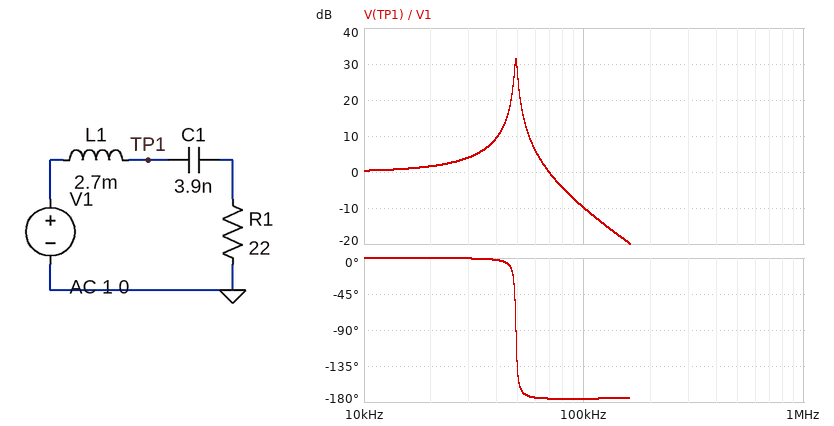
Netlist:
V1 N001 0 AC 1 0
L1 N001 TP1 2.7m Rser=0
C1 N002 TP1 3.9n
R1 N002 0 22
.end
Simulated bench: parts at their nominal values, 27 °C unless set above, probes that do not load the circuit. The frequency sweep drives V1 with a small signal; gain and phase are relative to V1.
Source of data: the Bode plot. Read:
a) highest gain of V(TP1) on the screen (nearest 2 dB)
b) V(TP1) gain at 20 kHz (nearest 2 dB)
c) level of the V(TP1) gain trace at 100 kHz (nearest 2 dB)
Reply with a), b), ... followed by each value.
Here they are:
a) 32 dB
b) 2 dB
c) -10 dB
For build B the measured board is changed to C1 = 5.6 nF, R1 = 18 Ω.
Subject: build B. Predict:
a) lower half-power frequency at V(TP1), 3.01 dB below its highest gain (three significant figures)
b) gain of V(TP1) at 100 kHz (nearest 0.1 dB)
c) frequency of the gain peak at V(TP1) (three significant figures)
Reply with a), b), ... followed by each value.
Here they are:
a) 40.4 kHz
b) -13.9 dB
c) 40.9 kHz
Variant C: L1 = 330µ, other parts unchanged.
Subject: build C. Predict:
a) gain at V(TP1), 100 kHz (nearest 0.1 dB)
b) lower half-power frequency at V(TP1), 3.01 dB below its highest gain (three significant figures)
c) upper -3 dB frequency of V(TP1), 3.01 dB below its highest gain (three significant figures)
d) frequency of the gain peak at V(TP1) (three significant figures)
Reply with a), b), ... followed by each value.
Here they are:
a) 6.1 dB
b) 135 kHz
c) 145 kHz
d) 140 kHz
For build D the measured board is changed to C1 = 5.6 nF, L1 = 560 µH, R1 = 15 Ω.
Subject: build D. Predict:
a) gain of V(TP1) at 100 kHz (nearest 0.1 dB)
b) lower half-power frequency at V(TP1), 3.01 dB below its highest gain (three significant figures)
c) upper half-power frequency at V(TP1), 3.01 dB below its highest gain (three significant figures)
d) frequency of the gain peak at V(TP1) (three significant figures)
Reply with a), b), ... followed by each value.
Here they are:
a) 12.3 dB
b) 87.7 kHz
c) 91.9 kHz
d) 89.8 kHz
